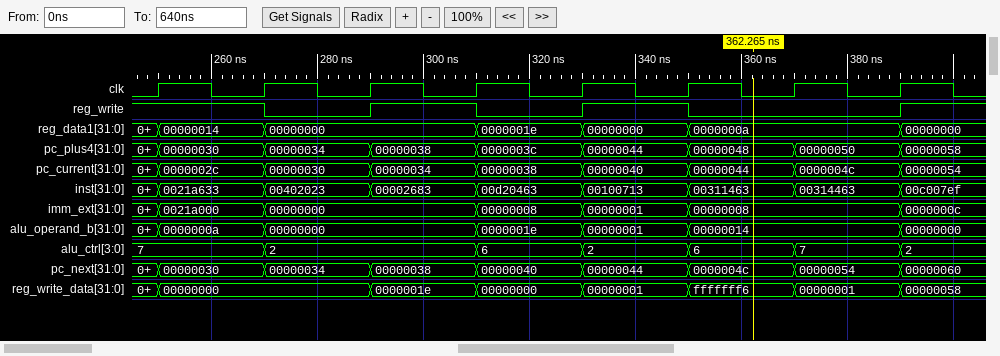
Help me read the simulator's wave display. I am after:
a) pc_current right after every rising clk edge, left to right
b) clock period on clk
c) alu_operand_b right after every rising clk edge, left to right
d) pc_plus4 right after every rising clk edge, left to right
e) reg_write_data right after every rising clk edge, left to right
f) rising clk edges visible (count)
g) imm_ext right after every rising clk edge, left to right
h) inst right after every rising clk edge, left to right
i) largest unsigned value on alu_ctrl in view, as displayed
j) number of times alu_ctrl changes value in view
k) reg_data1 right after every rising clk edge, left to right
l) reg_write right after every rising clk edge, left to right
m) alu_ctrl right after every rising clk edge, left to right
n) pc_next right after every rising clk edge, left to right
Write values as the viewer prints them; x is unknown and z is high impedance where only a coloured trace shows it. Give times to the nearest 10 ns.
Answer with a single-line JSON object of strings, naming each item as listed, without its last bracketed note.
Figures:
{"pc_current right after every rising clk edge, left to right": "0000002c, 00000030, 00000034, 00000038, 00000040, 00000044, 0000004c, 00000054", "clock period on clk": "20 ns", "alu_operand_b right after every rising clk edge, left to right": "0000000a, 00000000, 00000000, 0000001e, 00000001, 00000014, 00000014, 00000000", "pc_plus4 right after every rising clk edge, left to right": "00000030, 00000034, 00000038, 0000003c, 00000044, 00000048, 00000050, 00000058", "reg_write_data right after every rising clk edge, left to right": "00000000, 00000000, 0000001e, 00000000, 00000001, fffffff6, 00000001, 00000058", "rising clk edges visible": "8", "imm_ext right after every rising clk edge, left to right": "0021a000, 00000000, 00000000, 00000008, 00000001, 00000008, 00000008, 0000000c", "inst right after every rising clk edge, left to right": "0021a633, 00402023, 00002683, 00d20463, 00100713, 00311463, 00314463, 00c007ef", "largest unsigned value on alu_ctrl in view, as displayed": "7", "number of times alu_ctrl changes value in view": "6", "reg_data1 right after every rising clk edge, left to right": "00000014, 00000000, 00000000, 0000001e, 00000000, 0000000a, 0000000a, 00000000", "reg_write right after every rising clk edge, left to right": "1 0 1 0 1 0 0 1", "alu_ctrl right after every rising clk edge, left to right": "7, 2, 2, 6, 2, 6, 7, 2", "pc_next right after every rising clk edge, left to right": "00000030, 00000034, 00000038, 00000040, 00000044, 0000004c, 00000054, 00000060"}
